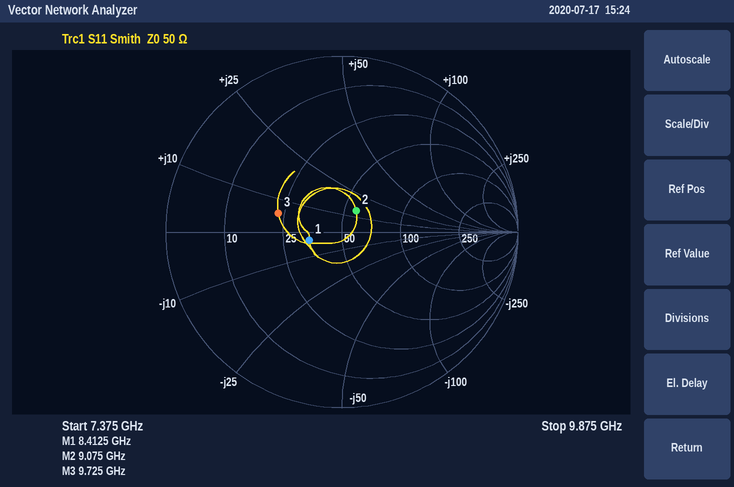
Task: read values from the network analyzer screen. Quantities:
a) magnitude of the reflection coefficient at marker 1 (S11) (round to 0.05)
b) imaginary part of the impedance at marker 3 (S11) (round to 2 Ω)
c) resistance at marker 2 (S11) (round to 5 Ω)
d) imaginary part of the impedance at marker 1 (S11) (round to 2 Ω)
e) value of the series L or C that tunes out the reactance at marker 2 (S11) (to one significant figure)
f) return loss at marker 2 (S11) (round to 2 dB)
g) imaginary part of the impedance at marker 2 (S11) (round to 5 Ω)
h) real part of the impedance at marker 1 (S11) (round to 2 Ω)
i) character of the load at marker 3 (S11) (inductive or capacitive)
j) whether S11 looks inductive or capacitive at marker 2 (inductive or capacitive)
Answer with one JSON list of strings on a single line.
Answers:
["0.20", "+6 Ω", "55 Ω", "-4 Ω", "1 pF", "16 dB", "+15 Ω", "34 Ω", "inductive", "inductive"]
